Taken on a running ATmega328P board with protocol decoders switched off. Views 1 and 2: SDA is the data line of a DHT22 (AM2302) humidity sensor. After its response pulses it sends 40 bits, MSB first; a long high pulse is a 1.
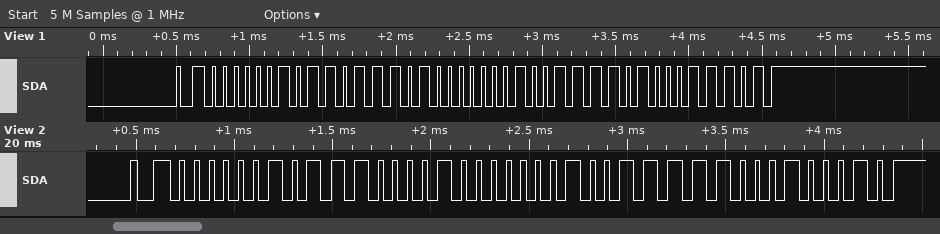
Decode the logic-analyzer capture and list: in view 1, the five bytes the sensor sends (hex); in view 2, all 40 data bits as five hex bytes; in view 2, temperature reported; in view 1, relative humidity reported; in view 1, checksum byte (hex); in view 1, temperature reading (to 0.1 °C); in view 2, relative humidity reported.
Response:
02 DD 01 3D 1D
02 E1 01 3E 22
31.8 °C
73.3 %
0x1D
31.7 °C
73.7 %
